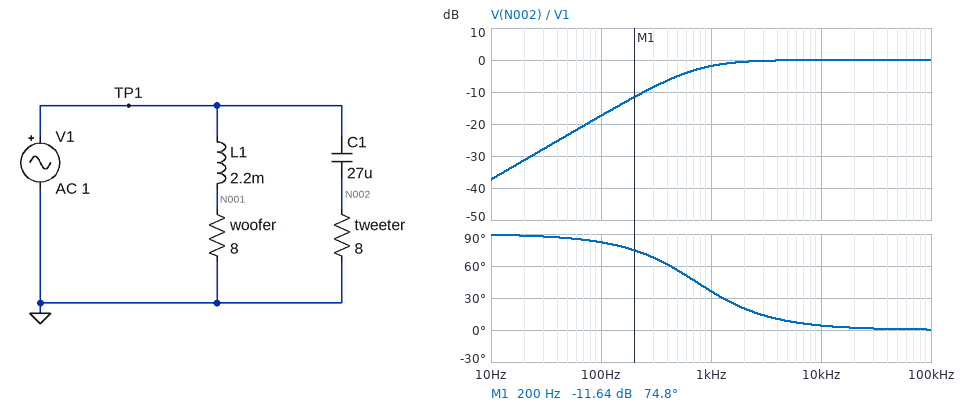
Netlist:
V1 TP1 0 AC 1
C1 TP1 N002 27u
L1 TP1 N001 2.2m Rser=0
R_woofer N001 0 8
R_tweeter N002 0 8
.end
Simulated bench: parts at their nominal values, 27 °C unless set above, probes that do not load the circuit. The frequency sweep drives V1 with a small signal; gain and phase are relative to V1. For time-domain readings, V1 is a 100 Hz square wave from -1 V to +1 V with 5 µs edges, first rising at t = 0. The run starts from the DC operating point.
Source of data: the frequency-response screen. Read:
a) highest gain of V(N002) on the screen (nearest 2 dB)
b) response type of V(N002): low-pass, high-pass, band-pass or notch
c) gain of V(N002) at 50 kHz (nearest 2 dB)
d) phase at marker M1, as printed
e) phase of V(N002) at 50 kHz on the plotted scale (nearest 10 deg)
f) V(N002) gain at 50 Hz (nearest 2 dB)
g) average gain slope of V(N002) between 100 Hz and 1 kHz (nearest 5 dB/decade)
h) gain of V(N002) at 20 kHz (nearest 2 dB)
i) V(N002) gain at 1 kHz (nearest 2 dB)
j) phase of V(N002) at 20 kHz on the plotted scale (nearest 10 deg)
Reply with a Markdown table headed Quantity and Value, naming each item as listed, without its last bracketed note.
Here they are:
| Quantity | Value |
|---|---|
| highest gain of V(N002) on the screen | 0 dB |
| response type of V(N002): low-pass, high-pass, band-pass or notch | high-pass |
| gain of V(N002) at 50 kHz | 0 dB |
| phase at marker M1, as printed | 74.8 deg |
| phase of V(N002) at 50 kHz on the plotted scale | 0 deg |
| V(N002) gain at 50 Hz | -24 dB |
| average gain slope of V(N002) between 100 Hz and 1 kHz | 15 dB/decade |
| gain of V(N002) at 20 kHz | 0 dB |
| V(N002) gain at 1 kHz | -2 dB |
| phase of V(N002) at 20 kHz on the plotted scale | 0 deg |
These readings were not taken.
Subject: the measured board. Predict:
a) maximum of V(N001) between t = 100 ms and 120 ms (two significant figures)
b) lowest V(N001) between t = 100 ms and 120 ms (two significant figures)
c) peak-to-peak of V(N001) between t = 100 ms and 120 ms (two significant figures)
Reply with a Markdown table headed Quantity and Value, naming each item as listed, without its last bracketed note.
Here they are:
| Quantity | Value |
|---|---|
| maximum of V(N001) between t = 100 ms and 120 ms | 1.0 V |
| lowest V(N001) between t = 100 ms and 120 ms | -1.0 V |
| peak-to-peak of V(N001) between t = 100 ms and 120 ms | 2.0 V |
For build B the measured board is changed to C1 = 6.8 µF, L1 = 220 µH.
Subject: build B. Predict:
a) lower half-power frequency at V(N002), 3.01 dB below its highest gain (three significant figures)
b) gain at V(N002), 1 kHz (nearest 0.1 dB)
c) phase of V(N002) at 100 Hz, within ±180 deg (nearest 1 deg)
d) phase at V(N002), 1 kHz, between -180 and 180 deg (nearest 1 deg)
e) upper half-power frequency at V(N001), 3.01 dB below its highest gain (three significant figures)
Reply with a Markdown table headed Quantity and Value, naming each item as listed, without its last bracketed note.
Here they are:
| Quantity | Value |
|---|---|
| lower half-power frequency at V(N002), 3.01 dB below its highest gain | 2.93 kHz |
| gain at V(N002), 1 kHz | -9.8 dB |
| phase of V(N002) at 100 Hz, within ±180 deg | 88 deg |
| phase at V(N002), 1 kHz, between -180 and 180 deg | 71 deg |
| upper half-power frequency at V(N001), 3.01 dB below its highest gain | 5.79 kHz |
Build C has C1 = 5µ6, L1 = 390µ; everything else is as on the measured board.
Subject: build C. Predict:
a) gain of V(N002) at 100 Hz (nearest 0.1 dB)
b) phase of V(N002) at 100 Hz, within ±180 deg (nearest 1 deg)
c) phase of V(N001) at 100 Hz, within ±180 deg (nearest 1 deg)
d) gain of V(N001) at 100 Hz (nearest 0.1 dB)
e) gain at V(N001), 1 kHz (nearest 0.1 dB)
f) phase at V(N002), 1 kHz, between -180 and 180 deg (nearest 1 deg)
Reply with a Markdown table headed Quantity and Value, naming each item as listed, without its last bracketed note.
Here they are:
| Quantity | Value |
|---|---|
| gain of V(N002) at 100 Hz | -31.0 dB |
| phase of V(N002) at 100 Hz, within ±180 deg | 88 deg |
| phase of V(N001) at 100 Hz, within ±180 deg | -2 deg |
| gain of V(N001) at 100 Hz | 0 dB |
| gain at V(N001), 1 kHz | -0.4 dB |
| phase at V(N002), 1 kHz, between -180 and 180 deg | 74 deg |
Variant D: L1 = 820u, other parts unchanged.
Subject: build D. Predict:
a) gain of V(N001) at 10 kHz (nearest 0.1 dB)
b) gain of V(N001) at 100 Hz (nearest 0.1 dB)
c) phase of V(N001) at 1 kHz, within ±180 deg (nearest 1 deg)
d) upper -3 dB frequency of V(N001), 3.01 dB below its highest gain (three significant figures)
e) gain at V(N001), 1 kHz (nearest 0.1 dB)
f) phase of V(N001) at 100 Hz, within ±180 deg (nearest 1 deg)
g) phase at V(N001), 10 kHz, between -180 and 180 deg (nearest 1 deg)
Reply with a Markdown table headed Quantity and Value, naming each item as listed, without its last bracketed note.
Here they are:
| Quantity | Value |
|---|---|
| gain of V(N001) at 10 kHz | -16.3 dB |
| gain of V(N001) at 100 Hz | 0 dB |
| phase of V(N001) at 1 kHz, within ±180 deg | -33 deg |
| upper -3 dB frequency of V(N001), 3.01 dB below its highest gain | 1.55 kHz |
| gain at V(N001), 1 kHz | -1.5 dB |
| phase of V(N001) at 100 Hz, within ±180 deg | -4 deg |
| phase at V(N001), 10 kHz, between -180 and 180 deg | -81 deg |
